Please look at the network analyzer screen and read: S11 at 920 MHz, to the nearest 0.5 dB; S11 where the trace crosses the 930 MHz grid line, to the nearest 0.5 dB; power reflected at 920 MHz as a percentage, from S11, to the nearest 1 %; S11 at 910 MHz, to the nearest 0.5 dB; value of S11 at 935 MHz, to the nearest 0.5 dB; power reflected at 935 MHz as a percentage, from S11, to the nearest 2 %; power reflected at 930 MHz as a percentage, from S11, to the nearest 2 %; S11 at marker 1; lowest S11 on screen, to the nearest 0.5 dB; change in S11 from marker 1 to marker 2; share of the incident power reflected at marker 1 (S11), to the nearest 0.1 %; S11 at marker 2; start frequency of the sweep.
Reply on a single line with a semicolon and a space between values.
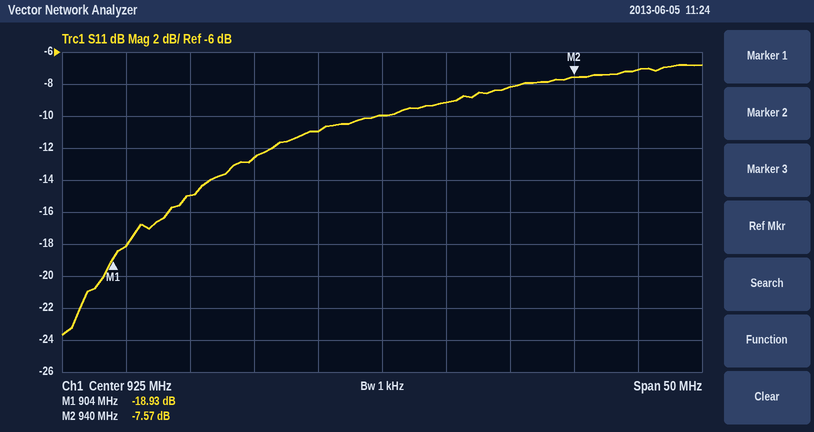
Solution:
-11.0 dB; -9.0 dB; 8 %; -15.0 dB; -8.0 dB; 16 %; 12 %; -18.93 dB; -23.5 dB; 11.36 dB; 1.3 %; -7.57 dB; 900 MHz
